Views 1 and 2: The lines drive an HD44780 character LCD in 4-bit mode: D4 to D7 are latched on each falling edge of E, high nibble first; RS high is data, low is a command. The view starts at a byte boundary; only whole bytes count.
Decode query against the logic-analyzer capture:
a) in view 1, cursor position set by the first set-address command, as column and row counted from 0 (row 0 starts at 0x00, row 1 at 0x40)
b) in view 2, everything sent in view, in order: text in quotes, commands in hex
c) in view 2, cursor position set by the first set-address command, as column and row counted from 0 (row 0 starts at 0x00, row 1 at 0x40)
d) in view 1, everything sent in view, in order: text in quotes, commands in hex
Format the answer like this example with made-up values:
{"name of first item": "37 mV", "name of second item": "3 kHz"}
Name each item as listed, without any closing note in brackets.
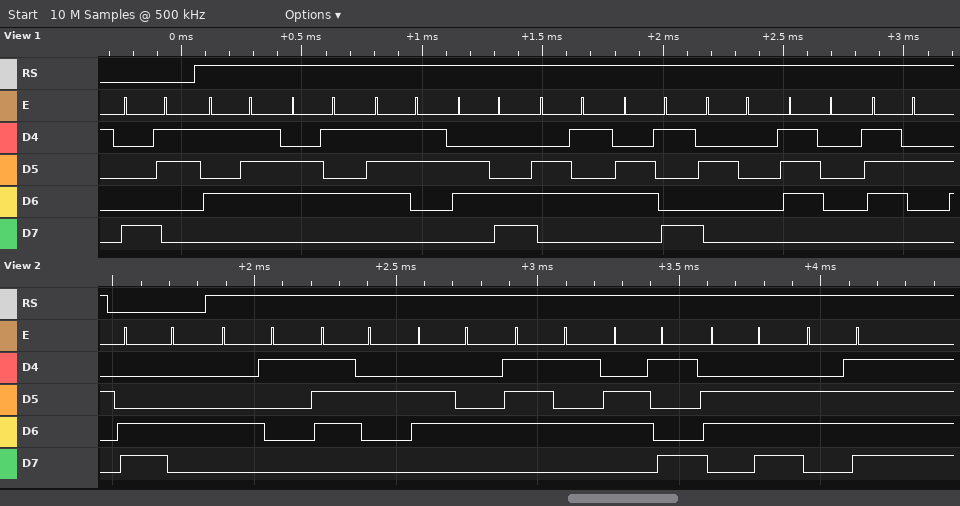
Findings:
{"in view 1, cursor position set by the first set-address command, as column and row counted from 0": "column 3, row 0", "in view 2, everything sent in view, in order: text in quotes, commands in hex": "0xC4 \"Arduino\"", "in view 2, cursor position set by the first set-address command, as column and row counted from 0": "column 4, row 1", "in view 1, everything sent in view, in order: text in quotes, commands in hex": "0x83 \"Weslei pr\""}
